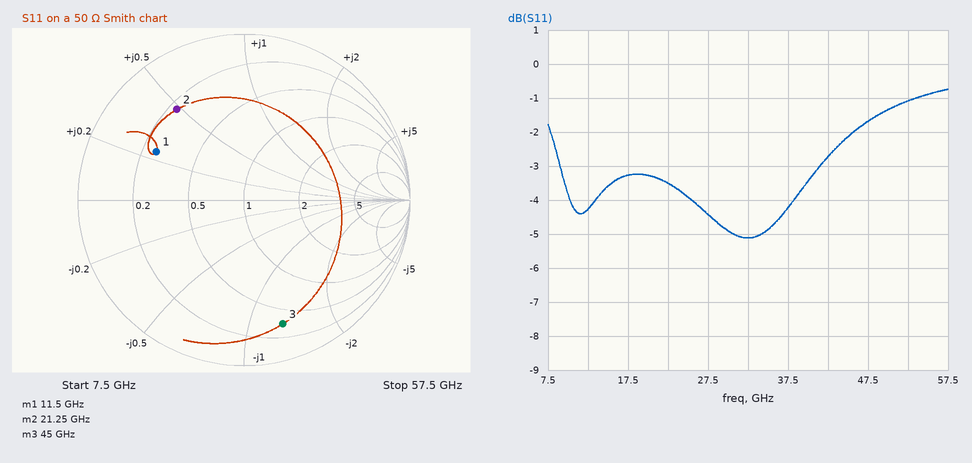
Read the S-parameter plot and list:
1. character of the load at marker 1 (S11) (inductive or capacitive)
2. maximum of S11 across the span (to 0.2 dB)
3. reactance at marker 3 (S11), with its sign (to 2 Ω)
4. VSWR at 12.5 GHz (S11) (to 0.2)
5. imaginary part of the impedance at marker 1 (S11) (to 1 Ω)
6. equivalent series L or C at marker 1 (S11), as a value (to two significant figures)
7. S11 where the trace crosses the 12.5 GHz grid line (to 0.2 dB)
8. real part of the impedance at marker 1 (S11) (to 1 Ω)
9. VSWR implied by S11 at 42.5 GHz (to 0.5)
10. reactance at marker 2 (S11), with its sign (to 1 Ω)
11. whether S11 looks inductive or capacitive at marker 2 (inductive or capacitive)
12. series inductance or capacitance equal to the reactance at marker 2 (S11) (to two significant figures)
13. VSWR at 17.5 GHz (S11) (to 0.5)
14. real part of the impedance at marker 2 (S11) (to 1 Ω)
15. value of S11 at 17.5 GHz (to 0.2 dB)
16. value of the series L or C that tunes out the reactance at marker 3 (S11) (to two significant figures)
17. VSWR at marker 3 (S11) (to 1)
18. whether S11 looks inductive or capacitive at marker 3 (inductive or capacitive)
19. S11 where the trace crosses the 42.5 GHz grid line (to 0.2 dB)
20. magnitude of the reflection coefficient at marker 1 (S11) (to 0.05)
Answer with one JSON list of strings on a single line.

["inductive", "-0.8 dB", "-66 Ω", "4.2", "+12 Ω", "170 pH", "-4.2 dB", "13 Ω", "6.5", "+24 Ω", "inductive", "180 pH", "5.5", "12 Ω", "-3.2 dB", "230 pH", "8", "capacitive", "-2.8 dB", "0.60"]
